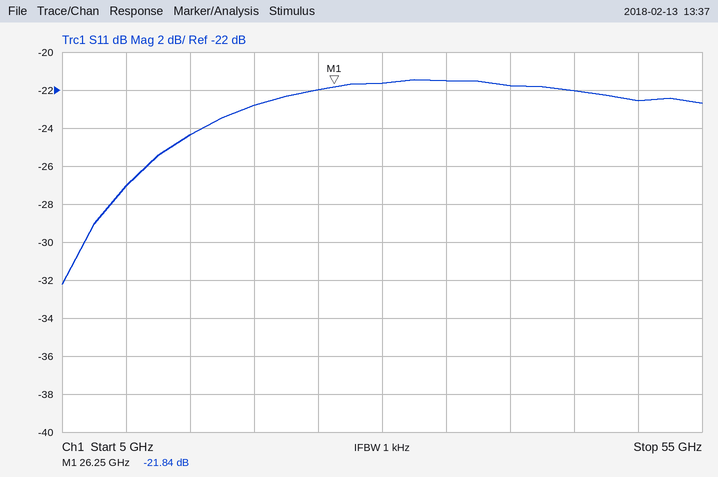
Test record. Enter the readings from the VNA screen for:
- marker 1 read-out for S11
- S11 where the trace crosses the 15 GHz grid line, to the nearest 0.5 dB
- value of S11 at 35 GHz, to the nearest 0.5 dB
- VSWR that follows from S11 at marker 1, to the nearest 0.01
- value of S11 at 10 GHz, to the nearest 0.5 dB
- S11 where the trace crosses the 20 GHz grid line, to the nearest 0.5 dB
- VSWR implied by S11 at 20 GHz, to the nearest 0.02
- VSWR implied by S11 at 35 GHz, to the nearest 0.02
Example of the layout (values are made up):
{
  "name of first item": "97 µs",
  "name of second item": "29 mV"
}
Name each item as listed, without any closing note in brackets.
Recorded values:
{
  "marker 1 read-out for S11": "-21.84 dB",
  "S11 where the trace crosses the 15 GHz grid line, to the nearest 0.5 dB": "-24.5 dB",
  "value of S11 at 35 GHz, to the nearest 0.5 dB": "-21.5 dB",
  "VSWR that follows from S11 at marker 1, to the nearest 0.01": "1.18",
  "value of S11 at 10 GHz, to the nearest 0.5 dB": "-27.0 dB",
  "S11 where the trace crosses the 20 GHz grid line, to the nearest 0.5 dB": "-23.0 dB",
  "VSWR implied by S11 at 20 GHz, to the nearest 0.02": "1.16",
  "VSWR implied by S11 at 35 GHz, to the nearest 0.02": "1.18"
}
